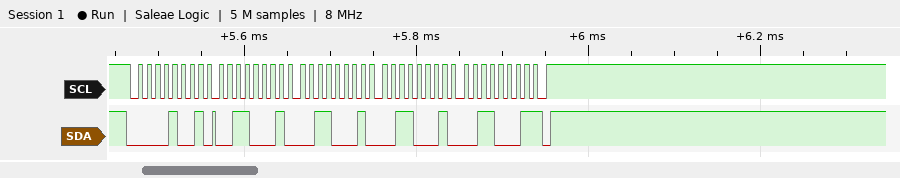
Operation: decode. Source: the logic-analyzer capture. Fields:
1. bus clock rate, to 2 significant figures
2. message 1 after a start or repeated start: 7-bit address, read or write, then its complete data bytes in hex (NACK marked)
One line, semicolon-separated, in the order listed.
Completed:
100 kHz; 0x04 read: 31 31 31 31 NACK
